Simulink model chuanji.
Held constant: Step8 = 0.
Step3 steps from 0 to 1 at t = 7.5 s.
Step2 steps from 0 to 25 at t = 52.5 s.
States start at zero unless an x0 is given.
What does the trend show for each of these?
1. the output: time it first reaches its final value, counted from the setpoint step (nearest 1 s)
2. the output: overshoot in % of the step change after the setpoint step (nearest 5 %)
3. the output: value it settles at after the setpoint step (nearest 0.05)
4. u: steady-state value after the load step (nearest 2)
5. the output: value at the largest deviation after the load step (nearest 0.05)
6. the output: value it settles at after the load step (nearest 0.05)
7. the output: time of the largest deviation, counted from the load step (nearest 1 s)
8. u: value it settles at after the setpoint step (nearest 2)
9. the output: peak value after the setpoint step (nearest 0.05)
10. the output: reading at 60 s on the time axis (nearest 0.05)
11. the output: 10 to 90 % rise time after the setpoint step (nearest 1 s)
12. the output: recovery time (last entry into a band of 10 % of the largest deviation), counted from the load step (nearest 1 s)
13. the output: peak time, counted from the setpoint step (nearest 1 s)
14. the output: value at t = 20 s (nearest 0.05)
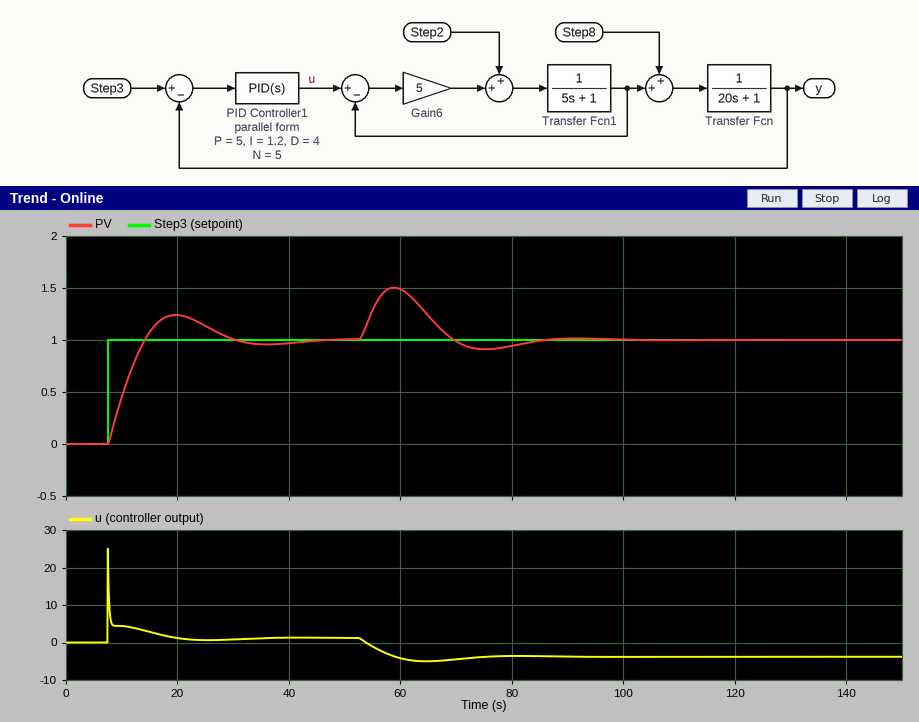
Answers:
7 s
25 %
1.00
-4
1.50
1.00
6 s
2
1.25
1.50
5 s
28 s
12 s
1.25
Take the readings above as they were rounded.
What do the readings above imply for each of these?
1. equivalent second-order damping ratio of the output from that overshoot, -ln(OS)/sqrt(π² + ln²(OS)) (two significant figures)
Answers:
0.40
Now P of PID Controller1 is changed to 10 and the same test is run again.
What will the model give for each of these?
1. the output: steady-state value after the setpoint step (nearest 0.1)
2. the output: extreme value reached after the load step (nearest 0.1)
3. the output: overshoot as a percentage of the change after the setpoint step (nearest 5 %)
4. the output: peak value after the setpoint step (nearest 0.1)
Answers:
1.0
1.4
10 %
1.1
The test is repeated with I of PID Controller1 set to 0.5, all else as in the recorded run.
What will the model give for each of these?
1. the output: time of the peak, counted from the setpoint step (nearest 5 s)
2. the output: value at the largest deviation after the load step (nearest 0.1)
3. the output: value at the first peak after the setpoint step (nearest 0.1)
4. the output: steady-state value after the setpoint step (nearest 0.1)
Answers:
20 s
1.6
1.1
1.0
